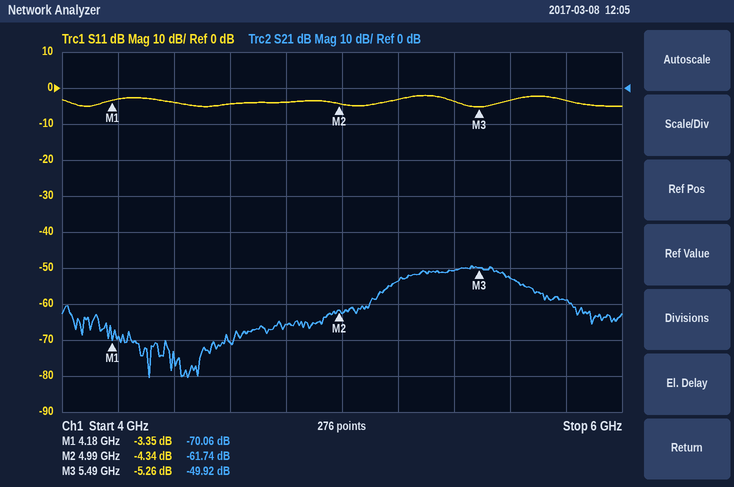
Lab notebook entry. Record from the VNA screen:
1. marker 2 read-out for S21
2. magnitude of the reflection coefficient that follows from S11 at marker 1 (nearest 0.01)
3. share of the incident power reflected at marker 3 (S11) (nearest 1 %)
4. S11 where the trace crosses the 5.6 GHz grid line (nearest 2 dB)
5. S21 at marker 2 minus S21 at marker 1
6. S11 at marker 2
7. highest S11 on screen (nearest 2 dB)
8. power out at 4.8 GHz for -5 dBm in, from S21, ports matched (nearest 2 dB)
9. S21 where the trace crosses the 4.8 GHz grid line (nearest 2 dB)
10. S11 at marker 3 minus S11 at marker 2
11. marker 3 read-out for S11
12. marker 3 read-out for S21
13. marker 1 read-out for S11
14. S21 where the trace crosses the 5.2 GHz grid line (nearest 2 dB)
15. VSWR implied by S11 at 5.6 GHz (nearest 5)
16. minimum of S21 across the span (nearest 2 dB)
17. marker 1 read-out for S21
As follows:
-61.74 dB
0.68
30 %
-4 dB
8.32 dB
-4.34 dB
-2 dB
-70 dBm
-66 dB
-0.92 dB
-5.26 dB
-49.92 dB
-3.35 dB
-54 dB
5
-80 dB
-70.06 dB
